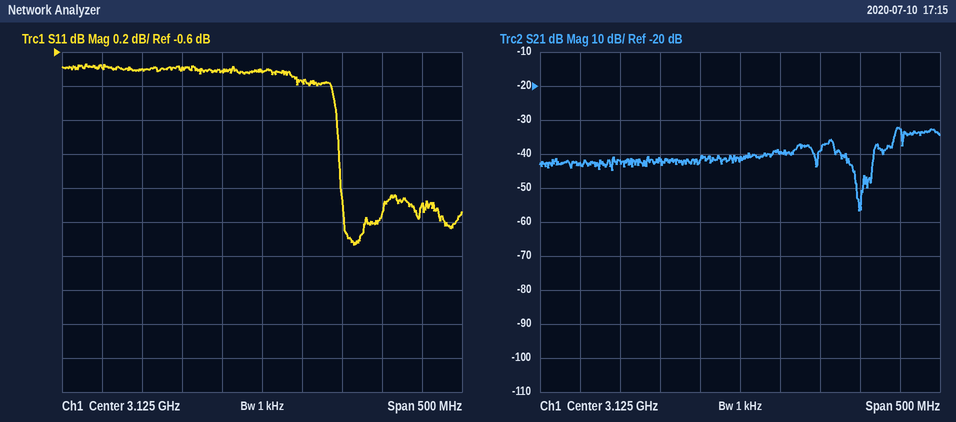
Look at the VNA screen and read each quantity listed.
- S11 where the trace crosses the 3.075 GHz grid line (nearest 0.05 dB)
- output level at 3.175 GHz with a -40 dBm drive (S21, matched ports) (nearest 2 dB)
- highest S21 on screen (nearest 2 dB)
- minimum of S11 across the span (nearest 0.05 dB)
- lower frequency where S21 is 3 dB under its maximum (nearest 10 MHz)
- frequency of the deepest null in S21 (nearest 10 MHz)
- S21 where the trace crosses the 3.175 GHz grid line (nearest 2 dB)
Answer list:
-0.70 dB
-80 dBm
-32 dB
-1.75 dB
3.32 GHz
3.27 GHz
-40 dB
